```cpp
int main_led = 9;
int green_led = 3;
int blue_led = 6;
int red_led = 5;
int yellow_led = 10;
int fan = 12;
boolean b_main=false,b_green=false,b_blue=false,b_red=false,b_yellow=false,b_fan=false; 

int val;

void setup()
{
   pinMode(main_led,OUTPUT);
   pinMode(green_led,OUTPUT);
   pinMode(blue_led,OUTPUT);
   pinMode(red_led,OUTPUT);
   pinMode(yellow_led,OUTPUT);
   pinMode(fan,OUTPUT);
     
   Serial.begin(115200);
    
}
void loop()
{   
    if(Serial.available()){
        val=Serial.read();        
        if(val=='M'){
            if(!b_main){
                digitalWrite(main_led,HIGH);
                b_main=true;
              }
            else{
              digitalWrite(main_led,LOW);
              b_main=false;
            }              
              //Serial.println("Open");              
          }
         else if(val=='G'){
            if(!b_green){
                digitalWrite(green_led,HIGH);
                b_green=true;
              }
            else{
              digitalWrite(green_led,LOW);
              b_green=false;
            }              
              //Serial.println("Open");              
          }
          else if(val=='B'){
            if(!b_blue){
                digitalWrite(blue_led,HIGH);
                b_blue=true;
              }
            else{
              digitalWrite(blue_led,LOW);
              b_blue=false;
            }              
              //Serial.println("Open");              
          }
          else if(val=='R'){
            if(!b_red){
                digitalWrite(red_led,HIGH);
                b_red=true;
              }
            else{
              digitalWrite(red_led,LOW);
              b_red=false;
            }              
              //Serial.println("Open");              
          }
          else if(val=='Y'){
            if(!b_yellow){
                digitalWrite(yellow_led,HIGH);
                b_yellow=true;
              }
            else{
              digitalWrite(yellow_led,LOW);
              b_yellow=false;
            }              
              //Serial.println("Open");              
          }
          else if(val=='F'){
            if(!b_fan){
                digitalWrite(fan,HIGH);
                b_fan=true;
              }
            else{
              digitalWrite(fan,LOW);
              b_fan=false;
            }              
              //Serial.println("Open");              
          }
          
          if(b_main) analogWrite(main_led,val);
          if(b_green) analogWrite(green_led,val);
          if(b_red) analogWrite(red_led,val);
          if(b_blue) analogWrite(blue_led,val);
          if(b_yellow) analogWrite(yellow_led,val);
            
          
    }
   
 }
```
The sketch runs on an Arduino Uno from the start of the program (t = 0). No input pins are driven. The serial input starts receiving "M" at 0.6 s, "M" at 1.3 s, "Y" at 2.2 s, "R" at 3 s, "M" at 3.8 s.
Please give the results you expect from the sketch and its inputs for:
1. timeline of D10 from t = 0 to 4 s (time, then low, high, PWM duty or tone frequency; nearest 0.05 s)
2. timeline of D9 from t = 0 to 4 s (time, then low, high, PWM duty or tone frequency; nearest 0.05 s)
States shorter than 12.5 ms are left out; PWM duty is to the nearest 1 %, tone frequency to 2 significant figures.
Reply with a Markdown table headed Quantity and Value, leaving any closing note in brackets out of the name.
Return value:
| Quantity | Value |
|---|---|
| timeline of D10 from t = 0 to 4 s | 0 s low; 2.2 s PWM 35 %; 3 s PWM 32 %; 3.8 s PWM 30 % |
| timeline of D9 from t = 0 to 4 s | 0 s low; 0.6 s PWM 30 %; 1.3 s low; 3.8 s PWM 30 % |
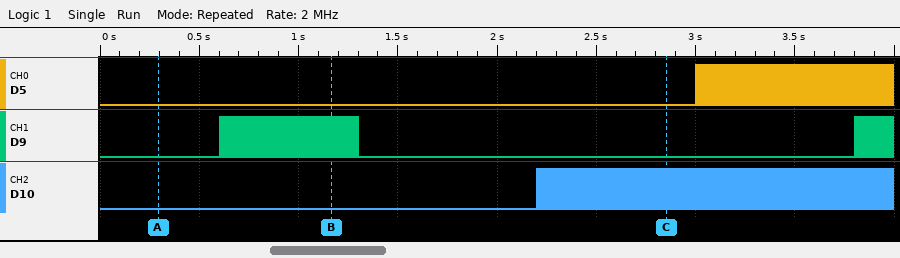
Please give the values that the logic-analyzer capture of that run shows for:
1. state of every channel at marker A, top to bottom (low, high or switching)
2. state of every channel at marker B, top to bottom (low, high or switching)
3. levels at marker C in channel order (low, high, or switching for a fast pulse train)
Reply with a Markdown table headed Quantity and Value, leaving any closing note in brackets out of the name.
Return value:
| Quantity | Value |
|---|---|
| state of every channel at marker A, top to bottom | D5 low, D9 low, D10 low |
| state of every channel at marker B, top to bottom | D5 low, D9 switching, D10 low |
| levels at marker C in channel order | D5 low, D9 low, D10 switching |
